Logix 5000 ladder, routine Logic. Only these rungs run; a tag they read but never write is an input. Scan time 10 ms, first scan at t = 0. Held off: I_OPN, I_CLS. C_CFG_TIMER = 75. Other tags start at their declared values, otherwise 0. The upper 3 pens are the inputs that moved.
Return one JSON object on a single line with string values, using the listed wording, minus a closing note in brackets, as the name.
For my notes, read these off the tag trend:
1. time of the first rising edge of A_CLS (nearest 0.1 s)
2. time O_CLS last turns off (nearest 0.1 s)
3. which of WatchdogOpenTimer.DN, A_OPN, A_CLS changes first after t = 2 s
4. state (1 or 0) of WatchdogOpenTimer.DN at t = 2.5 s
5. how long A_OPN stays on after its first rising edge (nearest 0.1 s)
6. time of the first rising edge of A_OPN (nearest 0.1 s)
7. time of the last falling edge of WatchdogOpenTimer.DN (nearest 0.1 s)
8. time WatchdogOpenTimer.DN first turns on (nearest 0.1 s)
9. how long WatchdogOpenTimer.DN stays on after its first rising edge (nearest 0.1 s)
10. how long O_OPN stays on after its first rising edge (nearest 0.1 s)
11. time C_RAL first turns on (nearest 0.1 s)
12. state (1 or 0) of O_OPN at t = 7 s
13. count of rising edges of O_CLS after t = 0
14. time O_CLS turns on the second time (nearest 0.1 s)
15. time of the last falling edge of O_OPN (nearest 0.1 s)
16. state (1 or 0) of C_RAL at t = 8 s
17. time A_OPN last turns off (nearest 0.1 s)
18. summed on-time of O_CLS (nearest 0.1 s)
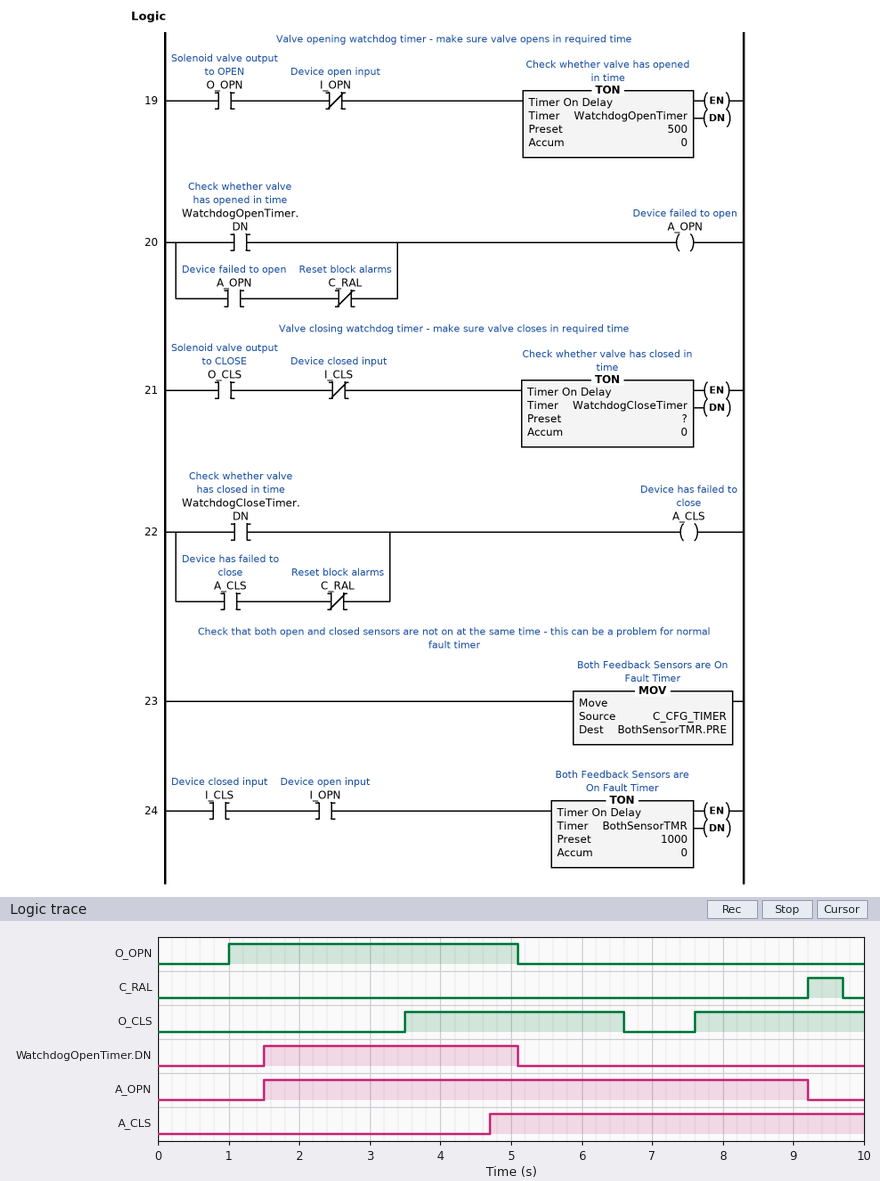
{"time of the first rising edge of A_CLS": "4.7 s", "time O_CLS last turns off": "6.6 s", "which of WatchdogOpenTimer.DN, A_OPN, A_CLS changes first after t = 2 s": "A_CLS", "state (1 or 0) of WatchdogOpenTimer.DN at t = 2.5 s": "1", "how long A_OPN stays on after its first rising edge": "7.7 s", "time of the first rising edge of A_OPN": "1.5 s", "time of the last falling edge of WatchdogOpenTimer.DN": "5.1 s", "time WatchdogOpenTimer.DN first turns on": "1.5 s", "how long WatchdogOpenTimer.DN stays on after its first rising edge": "3.6 s", "how long O_OPN stays on after its first rising edge": "4.1 s", "time C_RAL first turns on": "9.2 s", "state (1 or 0) of O_OPN at t = 7 s": "0", "count of rising edges of O_CLS after t = 0": "2", "time O_CLS turns on the second time": "7.6 s", "time of the last falling edge of O_OPN": "5.1 s", "state (1 or 0) of C_RAL at t = 8 s": "0", "time A_OPN last turns off": "9.2 s", "summed on-time of O_CLS": "5.5 s"}
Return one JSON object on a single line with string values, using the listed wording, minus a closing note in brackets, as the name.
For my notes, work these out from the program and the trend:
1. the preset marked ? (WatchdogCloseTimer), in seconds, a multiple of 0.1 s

{"the preset marked ? (WatchdogCloseTimer), in seconds, a multiple of 0.1 s": "1.2 s"}
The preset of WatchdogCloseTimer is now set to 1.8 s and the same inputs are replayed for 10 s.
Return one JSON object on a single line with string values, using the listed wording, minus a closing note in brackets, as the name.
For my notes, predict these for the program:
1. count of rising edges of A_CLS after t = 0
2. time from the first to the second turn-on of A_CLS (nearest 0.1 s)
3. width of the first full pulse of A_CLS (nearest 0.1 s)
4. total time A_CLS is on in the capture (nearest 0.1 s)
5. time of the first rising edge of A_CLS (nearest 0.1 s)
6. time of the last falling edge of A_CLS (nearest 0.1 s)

{"count of rising edges of A_CLS after t = 0": "2", "time from the first to the second turn-on of A_CLS": "4.1 s", "width of the first full pulse of A_CLS": "3.9 s", "total time A_CLS is on in the capture": "4.5 s", "time of the first rising edge of A_CLS": "5.3 s", "time of the last falling edge of A_CLS": "9.2 s"}
